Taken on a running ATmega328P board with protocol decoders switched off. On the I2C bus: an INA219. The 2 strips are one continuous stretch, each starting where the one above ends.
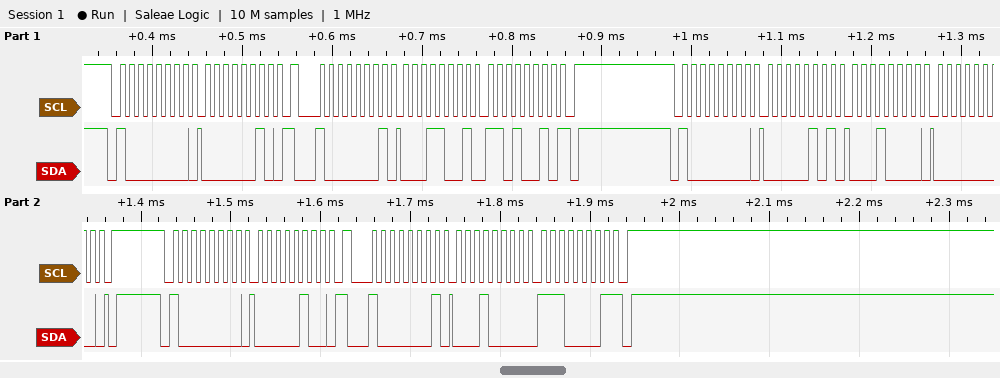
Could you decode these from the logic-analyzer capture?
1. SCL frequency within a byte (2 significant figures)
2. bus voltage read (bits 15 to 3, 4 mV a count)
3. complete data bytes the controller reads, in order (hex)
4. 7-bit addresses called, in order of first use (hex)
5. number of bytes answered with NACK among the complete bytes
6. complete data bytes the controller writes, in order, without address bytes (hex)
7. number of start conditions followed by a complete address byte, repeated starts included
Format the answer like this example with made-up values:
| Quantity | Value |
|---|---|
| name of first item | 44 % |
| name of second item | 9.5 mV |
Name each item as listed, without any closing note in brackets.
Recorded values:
| Quantity | Value |
|---|---|
| SCL frequency within a byte | 100 kHz |
| bus voltage read | 3.304 V |
| complete data bytes the controller reads, in order | 19 D2 10 E1 |
| 7-bit addresses called, in order of first use | 0x40 |
| number of bytes answered with NACK among the complete bytes | 2 |
| complete data bytes the controller writes, in order, without address bytes | 02 05 10 00 04 |
| number of start conditions followed by a complete address byte, repeated starts included | 5 |
